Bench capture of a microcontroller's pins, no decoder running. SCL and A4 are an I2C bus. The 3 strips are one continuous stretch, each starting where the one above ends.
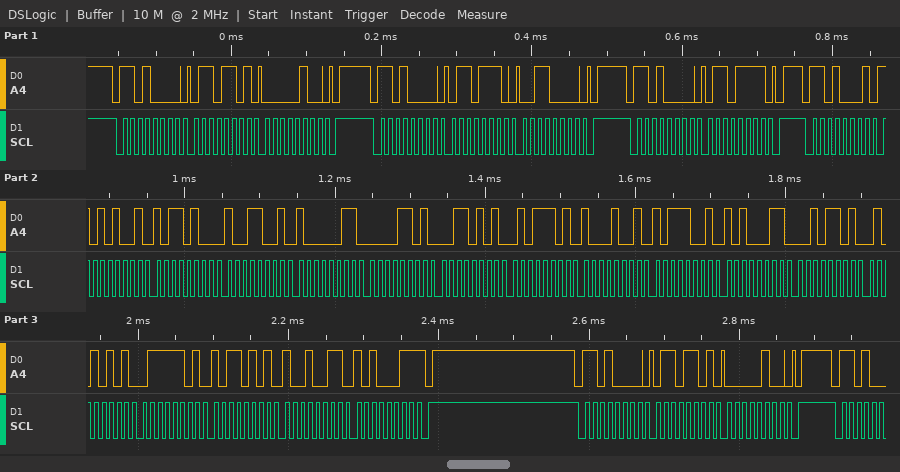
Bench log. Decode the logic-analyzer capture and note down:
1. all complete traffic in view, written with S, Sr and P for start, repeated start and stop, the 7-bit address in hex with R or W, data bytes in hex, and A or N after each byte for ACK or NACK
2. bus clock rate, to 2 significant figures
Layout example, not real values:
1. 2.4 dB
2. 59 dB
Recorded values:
1. S 68W A 6D A 04 A P S 68W A 6E A 30 A P S 68W A 6F A P S 68R A A9 A B4 A 99 A 83 A 0D A 35 A 5D A 89 A B9 A A3 A 2D A 55 A 7D A B5 A 93 A A3 N P S 68W A 6D A 04 A P
2. 100 kHz
